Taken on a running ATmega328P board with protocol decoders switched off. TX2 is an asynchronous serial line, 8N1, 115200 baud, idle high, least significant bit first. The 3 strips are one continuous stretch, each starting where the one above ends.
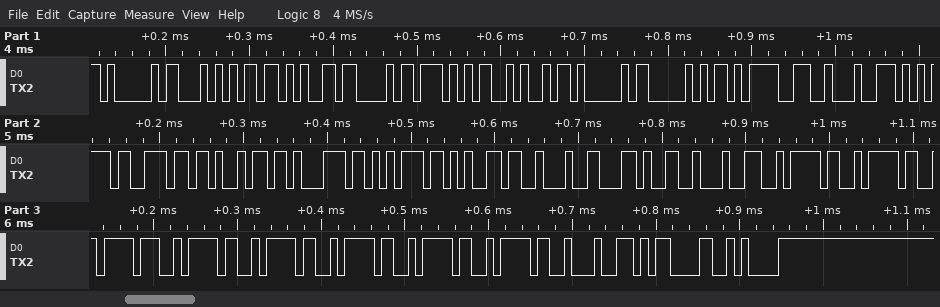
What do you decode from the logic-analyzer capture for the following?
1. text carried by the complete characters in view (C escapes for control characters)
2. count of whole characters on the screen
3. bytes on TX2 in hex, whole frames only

"AT+CWJAP=\"unique\",\"zzzzzzzz\"\r\n"
30
0x41 0x54 0x2B 0x43 0x57 0x4A 0x41 0x50 0x3D 0x22 0x75 0x6E 0x69 0x71 0x75 0x65 0x22 0x2C 0x22 0x7A 0x7A 0x7A 0x7A 0x7A 0x7A 0x7A 0x7A 0x22 0x0D 0x0A
